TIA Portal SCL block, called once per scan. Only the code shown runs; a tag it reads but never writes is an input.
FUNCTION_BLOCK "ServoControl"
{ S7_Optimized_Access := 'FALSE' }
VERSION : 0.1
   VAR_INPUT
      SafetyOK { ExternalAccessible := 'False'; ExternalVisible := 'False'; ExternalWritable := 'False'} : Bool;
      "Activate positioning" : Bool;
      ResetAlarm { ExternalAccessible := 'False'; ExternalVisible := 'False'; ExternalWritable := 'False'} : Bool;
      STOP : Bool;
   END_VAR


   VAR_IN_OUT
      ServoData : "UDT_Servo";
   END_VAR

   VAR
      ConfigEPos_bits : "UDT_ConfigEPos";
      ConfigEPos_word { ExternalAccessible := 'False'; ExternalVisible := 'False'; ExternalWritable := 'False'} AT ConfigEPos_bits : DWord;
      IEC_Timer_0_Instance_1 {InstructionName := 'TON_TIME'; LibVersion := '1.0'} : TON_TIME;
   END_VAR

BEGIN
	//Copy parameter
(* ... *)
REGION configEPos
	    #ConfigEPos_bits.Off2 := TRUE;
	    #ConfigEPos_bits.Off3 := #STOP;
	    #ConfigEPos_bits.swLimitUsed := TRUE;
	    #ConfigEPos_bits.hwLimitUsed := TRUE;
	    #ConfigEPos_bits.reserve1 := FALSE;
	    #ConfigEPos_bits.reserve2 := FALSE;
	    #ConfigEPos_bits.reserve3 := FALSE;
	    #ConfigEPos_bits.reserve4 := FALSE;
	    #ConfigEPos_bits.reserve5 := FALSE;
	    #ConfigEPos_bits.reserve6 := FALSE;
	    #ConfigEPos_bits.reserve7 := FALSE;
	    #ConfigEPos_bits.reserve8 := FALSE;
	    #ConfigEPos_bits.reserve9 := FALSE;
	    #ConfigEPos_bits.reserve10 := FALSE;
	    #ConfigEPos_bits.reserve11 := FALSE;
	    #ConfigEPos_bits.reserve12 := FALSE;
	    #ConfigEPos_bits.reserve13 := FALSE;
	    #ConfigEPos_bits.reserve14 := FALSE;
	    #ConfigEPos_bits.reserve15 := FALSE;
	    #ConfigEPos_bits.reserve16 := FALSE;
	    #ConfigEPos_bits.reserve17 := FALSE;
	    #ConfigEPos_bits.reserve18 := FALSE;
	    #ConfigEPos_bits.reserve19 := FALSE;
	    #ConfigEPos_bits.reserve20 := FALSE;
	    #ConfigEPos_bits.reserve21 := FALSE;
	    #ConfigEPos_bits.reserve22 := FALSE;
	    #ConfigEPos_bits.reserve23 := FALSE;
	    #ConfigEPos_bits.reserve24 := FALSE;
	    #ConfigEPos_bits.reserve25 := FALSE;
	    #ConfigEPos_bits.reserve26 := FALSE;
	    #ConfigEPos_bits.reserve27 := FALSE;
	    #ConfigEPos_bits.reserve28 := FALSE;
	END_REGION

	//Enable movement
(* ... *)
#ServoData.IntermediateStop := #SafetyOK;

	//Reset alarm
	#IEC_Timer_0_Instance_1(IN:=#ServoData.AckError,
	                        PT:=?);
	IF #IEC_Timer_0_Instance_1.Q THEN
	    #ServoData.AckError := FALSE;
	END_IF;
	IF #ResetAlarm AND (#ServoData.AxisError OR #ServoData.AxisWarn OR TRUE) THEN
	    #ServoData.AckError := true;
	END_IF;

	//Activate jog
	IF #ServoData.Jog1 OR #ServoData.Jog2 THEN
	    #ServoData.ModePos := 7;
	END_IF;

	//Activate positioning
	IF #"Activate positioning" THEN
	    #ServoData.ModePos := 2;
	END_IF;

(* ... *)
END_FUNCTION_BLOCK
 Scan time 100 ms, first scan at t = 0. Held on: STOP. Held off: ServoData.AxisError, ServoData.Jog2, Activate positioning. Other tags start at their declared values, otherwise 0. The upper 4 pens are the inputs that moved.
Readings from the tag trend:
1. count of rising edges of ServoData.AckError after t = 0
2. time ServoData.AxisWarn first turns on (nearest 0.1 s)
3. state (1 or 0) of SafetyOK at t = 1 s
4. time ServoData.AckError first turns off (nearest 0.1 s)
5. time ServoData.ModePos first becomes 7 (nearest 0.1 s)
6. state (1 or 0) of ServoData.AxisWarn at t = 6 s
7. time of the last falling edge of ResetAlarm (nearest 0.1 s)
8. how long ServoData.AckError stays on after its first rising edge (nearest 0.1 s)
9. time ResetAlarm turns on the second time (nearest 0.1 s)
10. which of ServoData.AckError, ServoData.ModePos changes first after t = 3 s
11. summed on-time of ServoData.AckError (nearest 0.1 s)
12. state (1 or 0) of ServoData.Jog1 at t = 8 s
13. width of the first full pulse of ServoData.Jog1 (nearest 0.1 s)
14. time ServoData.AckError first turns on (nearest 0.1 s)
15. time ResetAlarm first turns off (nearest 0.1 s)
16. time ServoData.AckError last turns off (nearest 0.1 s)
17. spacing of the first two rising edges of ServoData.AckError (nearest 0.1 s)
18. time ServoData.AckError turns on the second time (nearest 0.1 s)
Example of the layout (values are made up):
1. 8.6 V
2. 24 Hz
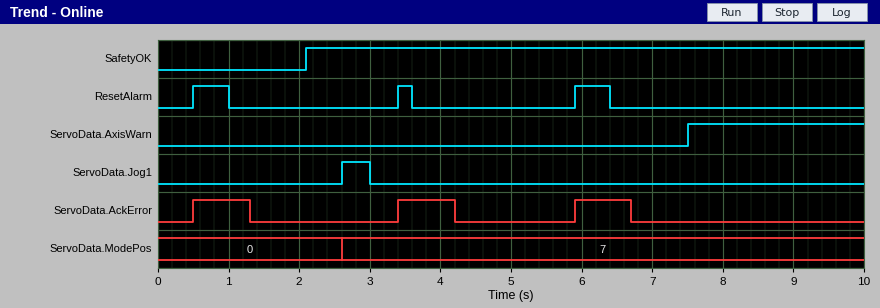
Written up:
1. 3
2. 7.5 s
3. 0
4. 1.3 s
5. 2.6 s
6. 0
7. 6.4 s
8. 0.8 s
9. 3.4 s
10. ServoData.AckError
11. 2.4 s
12. 0
13. 0.4 s
14. 0.5 s
15. 1.0 s
16. 6.7 s
17. 2.9 s
18. 3.4 s
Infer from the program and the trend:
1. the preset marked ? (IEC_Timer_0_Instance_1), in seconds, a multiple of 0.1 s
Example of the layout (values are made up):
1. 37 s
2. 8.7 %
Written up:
1. 0.7 s
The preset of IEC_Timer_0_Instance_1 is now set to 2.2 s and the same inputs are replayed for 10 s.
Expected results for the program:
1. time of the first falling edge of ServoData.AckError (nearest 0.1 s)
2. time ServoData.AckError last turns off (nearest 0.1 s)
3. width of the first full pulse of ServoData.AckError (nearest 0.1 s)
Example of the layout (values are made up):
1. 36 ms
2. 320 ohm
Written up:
1. 2.8 s
2. 8.2 s
3. 2.3 s
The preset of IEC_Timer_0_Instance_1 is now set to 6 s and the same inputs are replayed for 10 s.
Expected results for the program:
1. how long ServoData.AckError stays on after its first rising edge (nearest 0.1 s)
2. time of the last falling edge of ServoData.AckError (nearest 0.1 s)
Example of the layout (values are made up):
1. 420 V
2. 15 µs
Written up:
1. 6.1 s
2. 6.6 s
